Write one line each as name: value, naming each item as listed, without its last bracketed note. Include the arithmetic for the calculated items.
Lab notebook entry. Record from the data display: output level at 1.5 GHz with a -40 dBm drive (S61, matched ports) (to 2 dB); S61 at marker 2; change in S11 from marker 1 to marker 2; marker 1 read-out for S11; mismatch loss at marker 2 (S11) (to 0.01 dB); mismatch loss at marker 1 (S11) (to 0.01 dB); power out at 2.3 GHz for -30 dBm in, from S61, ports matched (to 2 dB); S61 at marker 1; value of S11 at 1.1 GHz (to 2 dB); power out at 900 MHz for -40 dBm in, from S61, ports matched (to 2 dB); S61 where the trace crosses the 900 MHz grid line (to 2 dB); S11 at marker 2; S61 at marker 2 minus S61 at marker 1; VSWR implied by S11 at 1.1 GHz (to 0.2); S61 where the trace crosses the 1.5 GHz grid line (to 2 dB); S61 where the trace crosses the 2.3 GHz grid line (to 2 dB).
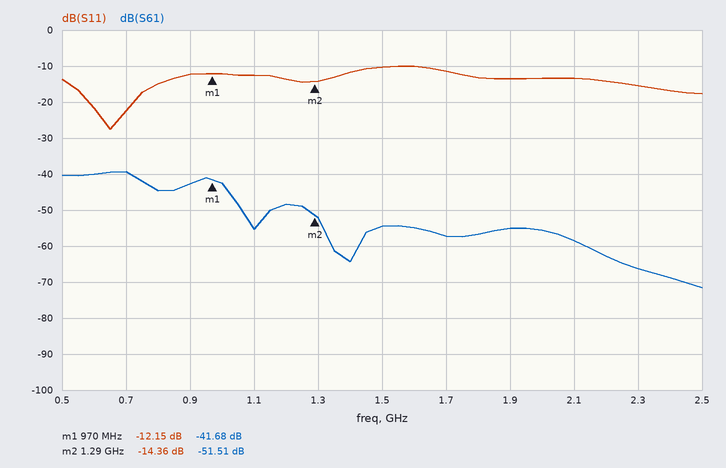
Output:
output level at 1.5 GHz with a -40 dBm drive (S61, matched ports): -40 dBm + (-54 dB) = -94 dBm
S61 at marker 2: -51.51 dB
change in S11 from marker 1 to marker 2: -14.36 − (-12.15) = -2.21 dB
marker 1 read-out for S11: -12.15 dB
mismatch loss at marker 2 (S11): −10 log10(1 − 10^(-14.36/10)) ≈ 0.16 dB
mismatch loss at marker 1 (S11): −10 log10(1 − 10^(-12.15/10)) ≈ 0.27 dB
power out at 2.3 GHz for -30 dBm in, from S61, ports matched: -30 dBm + (-66 dB) = -96 dBm
S61 at marker 1: -41.68 dB
value of S11 at 1.1 GHz: -12 dB
power out at 900 MHz for -40 dBm in, from S61, ports matched: -40 dBm + (-42 dB) = -82 dBm
S61 where the trace crosses the 900 MHz grid line: -42 dB
S11 at marker 2: -14.36 dB
S61 at marker 2 minus S61 at marker 1: -51.51 − (-41.68) = -9.83 dB
VSWR implied by S11 at 1.1 GHz: |Γ| = 10^(-12/20) = 0.2512; VSWR = (1 + 0.2512)/(1 − 0.2512) ≈ 1.67, so 1.6 to the nearest 0.2
S61 where the trace crosses the 1.5 GHz grid line: -54 dB
S61 where the trace crosses the 2.3 GHz grid line: -66 dB
